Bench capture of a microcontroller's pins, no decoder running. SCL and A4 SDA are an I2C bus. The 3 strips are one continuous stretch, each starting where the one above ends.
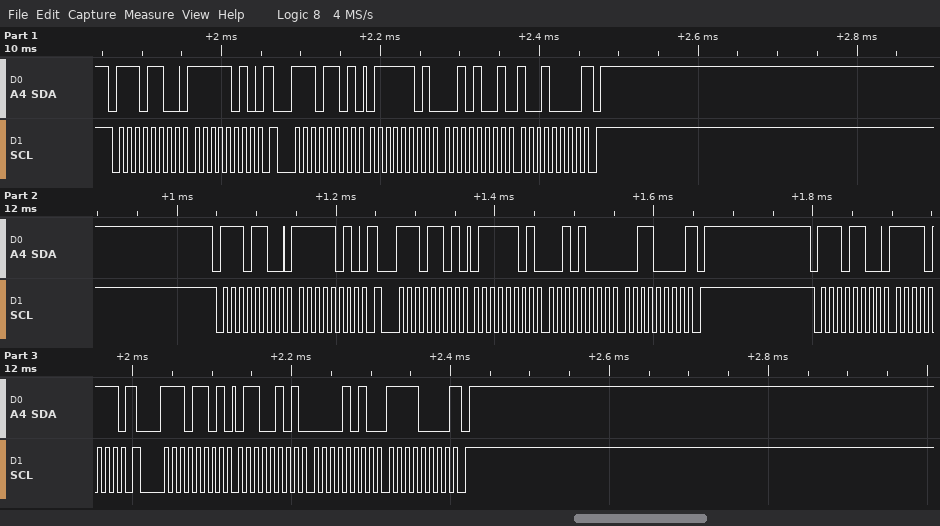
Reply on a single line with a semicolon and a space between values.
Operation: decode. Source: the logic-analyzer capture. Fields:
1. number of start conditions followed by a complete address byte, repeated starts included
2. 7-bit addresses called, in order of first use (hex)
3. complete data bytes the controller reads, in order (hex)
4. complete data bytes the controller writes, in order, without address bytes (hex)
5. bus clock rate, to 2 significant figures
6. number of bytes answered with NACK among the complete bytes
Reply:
6; 0x76; 7D 29 90 7D 28 30 65 0A F0; FA FA F7; 100 kHz; 3
